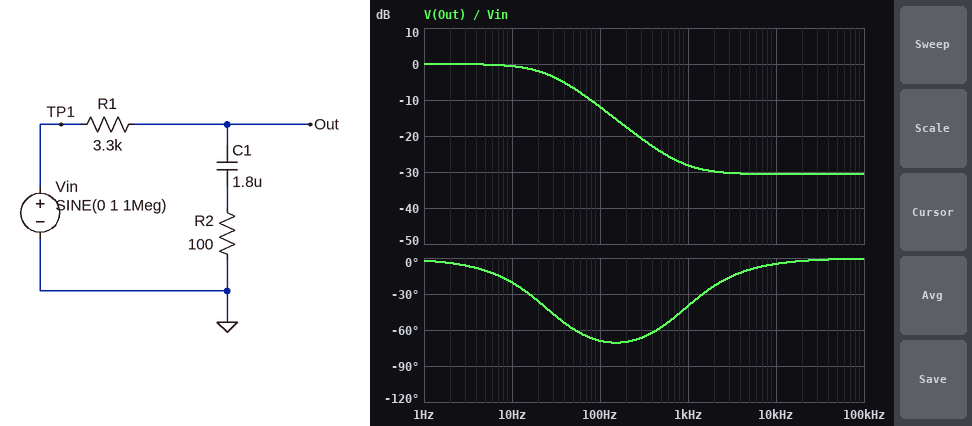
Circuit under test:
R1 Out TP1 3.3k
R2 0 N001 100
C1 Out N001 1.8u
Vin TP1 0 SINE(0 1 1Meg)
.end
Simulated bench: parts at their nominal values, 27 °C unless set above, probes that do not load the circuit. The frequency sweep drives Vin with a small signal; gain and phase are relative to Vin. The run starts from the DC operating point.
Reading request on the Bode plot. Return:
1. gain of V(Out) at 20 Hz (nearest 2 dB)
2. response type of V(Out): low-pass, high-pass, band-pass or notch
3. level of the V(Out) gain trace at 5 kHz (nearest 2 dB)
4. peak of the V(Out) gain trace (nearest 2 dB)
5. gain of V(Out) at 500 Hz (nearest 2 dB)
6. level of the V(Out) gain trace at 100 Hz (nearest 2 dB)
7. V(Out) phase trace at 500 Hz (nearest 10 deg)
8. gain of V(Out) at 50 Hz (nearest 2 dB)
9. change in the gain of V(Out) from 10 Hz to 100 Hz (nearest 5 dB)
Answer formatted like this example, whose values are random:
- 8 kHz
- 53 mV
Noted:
- -2 dB
- low-pass
- -30 dB
- 0 dB
- -24 dB
- -12 dB
- -60 deg
- -6 dB
- -10 dB
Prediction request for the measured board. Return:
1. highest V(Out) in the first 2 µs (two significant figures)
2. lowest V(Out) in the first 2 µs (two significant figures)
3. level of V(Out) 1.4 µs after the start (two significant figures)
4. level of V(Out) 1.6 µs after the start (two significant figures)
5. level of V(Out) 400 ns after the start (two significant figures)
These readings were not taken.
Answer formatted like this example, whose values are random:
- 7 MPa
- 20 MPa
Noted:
- 29 mV
- -29 mV
- 17 mV
- -17 mV
- 17 mV
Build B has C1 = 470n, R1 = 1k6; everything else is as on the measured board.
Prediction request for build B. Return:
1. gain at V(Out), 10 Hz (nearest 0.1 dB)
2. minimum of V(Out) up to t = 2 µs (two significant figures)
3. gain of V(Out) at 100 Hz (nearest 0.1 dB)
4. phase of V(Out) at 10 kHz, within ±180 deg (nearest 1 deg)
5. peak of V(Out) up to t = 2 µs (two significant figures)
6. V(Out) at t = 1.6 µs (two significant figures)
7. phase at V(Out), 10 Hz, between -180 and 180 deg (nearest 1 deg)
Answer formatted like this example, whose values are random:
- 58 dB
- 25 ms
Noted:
- 0 dB
- -59 mV
- -1.0 dB
- -18 deg
- 59 mV
- -34 mV
- -3 deg
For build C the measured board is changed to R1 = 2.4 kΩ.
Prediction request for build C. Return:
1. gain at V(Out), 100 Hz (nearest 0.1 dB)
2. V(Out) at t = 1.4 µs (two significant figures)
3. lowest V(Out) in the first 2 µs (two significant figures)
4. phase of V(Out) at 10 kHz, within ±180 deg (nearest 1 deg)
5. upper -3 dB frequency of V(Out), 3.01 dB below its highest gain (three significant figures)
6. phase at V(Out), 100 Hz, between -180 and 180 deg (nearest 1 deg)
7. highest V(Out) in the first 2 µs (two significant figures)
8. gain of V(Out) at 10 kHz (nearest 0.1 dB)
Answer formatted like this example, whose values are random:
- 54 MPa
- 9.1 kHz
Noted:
- -9.5 dB
- 24 mV
- -40 mV
- -5 deg
- 35.4 Hz
- -64 deg
- 40 mV
- -27.9 dB
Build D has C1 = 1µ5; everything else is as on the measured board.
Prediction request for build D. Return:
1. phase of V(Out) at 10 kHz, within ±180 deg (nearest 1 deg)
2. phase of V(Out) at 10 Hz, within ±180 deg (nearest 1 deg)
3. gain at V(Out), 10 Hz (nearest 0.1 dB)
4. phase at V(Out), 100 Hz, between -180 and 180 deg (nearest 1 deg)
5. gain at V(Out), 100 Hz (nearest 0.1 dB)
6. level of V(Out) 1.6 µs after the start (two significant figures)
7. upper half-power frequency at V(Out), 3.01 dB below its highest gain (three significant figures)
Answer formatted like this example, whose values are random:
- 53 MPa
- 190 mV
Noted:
- -6 deg
- -17 deg
- -0.4 dB
- -67 deg
- -10.5 dB
- -17 mV
- 31.2 Hz
